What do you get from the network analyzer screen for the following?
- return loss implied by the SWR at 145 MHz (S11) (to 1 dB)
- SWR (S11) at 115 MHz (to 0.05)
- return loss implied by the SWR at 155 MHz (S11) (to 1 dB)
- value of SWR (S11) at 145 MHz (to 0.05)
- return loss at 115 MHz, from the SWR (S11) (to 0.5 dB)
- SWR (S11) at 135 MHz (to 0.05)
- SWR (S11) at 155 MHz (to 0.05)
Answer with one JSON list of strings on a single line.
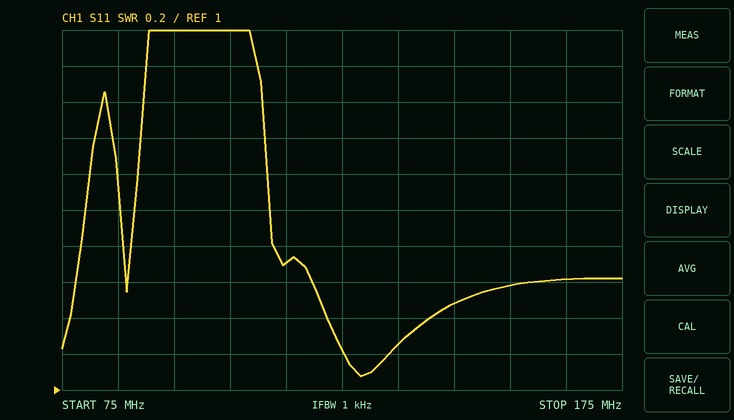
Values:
["14 dB", "1.70", "13 dB", "1.50", "11.5 dB", "1.25", "1.60"]
